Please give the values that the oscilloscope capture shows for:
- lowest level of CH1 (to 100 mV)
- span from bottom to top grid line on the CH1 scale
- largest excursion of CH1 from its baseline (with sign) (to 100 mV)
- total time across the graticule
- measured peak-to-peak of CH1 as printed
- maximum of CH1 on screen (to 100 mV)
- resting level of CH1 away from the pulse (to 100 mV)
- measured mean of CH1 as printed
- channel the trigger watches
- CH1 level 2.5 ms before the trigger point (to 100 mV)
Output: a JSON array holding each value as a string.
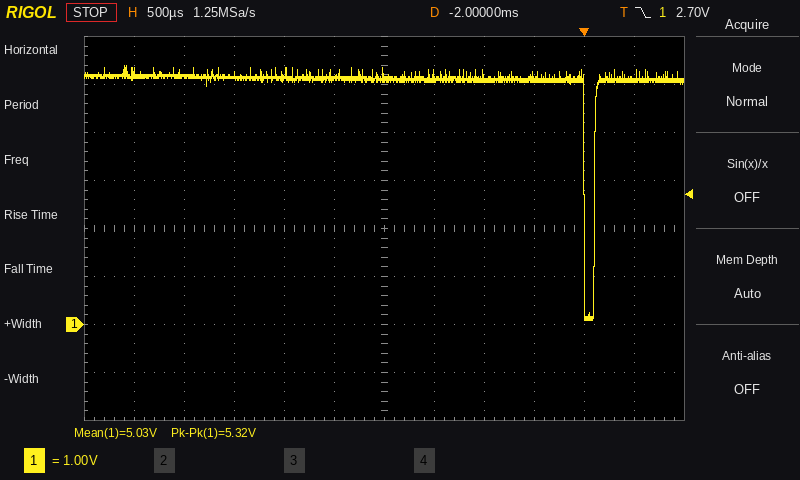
["100 mV", "8 V", "-5.0 V", "6 ms", "5.32 V", "5.4 V", "5.1 V", "5.03 V", "CH1", "5.1 V"]
